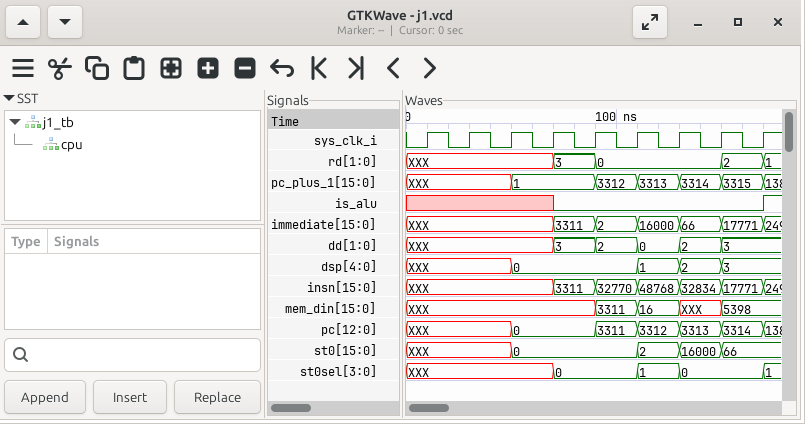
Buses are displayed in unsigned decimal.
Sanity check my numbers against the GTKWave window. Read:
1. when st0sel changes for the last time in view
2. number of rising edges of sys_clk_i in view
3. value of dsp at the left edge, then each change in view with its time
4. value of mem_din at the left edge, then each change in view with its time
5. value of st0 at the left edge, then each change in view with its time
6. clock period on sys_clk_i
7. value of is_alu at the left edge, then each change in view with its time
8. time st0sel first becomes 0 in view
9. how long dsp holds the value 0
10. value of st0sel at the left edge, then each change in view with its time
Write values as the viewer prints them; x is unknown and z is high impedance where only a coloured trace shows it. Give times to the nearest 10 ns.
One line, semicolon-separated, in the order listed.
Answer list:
170 ns; 9; XXX, 0 at 50 ns, 1 at 110 ns, 2 at 130 ns, 3 at 150 ns; XXX, 3311 at 90 ns, 16 at 110 ns, XXX at 130 ns, 5398 at 150 ns; XXX, 0 at 50 ns, 2 at 110 ns, 16000 at 130 ns, 66 at 150 ns; 20 ns; x, 0 at 70 ns, 1 at 170 ns; 70 ns; 60 ns; XXX, 0 at 70 ns, 1 at 110 ns, 0 at 130 ns, 1 at 170 ns
